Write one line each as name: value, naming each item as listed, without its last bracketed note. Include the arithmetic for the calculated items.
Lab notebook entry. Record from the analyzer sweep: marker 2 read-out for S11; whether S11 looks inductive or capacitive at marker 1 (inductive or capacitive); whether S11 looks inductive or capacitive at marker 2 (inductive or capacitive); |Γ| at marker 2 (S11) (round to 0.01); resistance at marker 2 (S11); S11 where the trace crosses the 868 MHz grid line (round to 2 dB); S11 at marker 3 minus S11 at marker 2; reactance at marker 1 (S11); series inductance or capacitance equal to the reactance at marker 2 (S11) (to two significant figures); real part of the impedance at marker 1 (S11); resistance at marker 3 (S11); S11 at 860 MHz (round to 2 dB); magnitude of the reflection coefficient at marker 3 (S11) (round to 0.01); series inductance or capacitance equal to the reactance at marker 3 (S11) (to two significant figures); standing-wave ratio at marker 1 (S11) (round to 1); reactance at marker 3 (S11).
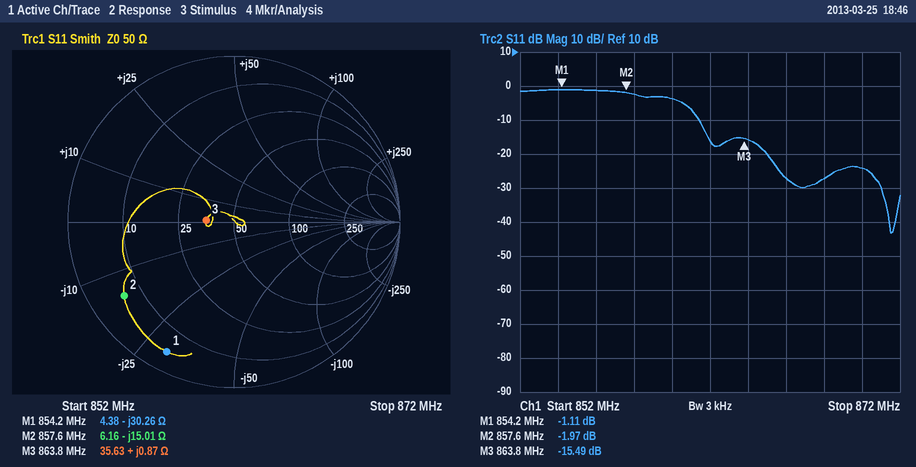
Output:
marker 2 read-out for S11: -1.97 dB
whether S11 looks inductive or capacitive at marker 1: capacitive
whether S11 looks inductive or capacitive at marker 2: capacitive
|Γ| at marker 2 (S11): 0.80
resistance at marker 2: 6.16 Ω
S11 where the trace crosses the 868 MHz grid line: -28 dB
S11 at marker 3 minus S11 at marker 2: -15.49 − (-1.97) = -13.52 dB
reactance at marker 1: -30.26 Ω
series inductance or capacitance equal to the reactance at marker 2 (S11): C = 1/(2π × 857.6 MHz × 15.01 Ω) ≈ 12 pF
real part of the impedance at marker 1: 4.38 Ω
resistance at marker 3: 35.63 Ω
S11 at 860 MHz: -4 dB
magnitude of the reflection coefficient at marker 3 (S11): 0.17
series inductance or capacitance equal to the reactance at marker 3 (S11): L = 0.87 Ω/(2π × 863.8 MHz) ≈ 160 pH
standing-wave ratio at marker 1 (S11): 16
reactance at marker 3: +0.87 Ω
